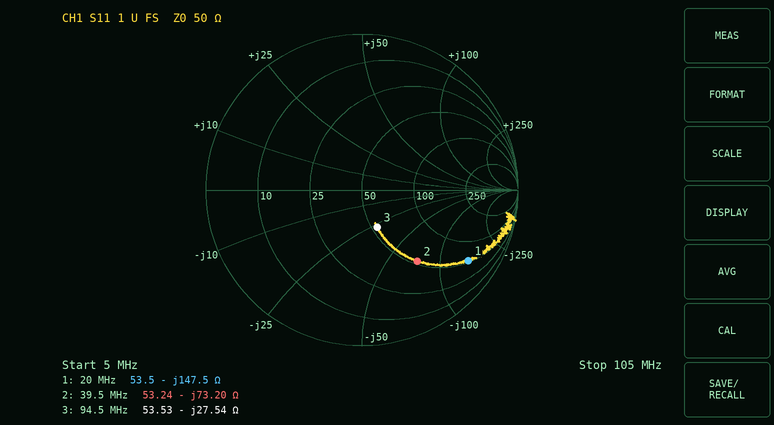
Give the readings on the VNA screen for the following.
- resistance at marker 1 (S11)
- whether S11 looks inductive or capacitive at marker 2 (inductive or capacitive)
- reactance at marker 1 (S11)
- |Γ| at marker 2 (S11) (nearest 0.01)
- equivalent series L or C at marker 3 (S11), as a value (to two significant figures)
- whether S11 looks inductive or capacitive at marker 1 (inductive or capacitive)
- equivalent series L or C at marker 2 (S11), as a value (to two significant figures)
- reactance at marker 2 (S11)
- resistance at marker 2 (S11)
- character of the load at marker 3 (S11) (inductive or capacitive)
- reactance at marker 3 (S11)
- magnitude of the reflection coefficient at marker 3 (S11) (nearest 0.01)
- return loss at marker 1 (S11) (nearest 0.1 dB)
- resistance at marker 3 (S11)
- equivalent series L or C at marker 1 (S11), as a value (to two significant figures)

53.5 Ω
capacitive
-147.5 Ω
0.58
61 pF
capacitive
55 pF
-73.20 Ω
53.24 Ω
capacitive
-27.54 Ω
0.26
1.7 dB
53.53 Ω
54 pF
